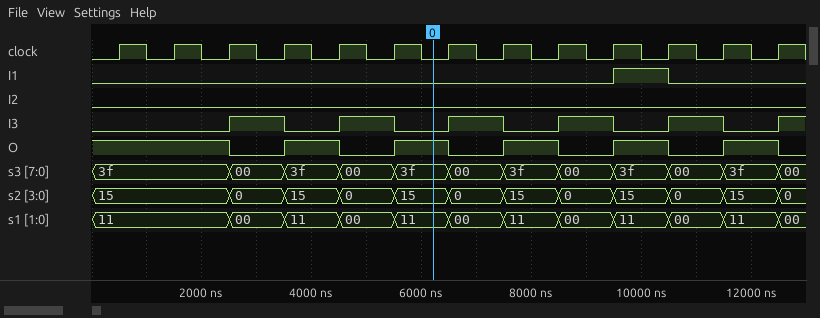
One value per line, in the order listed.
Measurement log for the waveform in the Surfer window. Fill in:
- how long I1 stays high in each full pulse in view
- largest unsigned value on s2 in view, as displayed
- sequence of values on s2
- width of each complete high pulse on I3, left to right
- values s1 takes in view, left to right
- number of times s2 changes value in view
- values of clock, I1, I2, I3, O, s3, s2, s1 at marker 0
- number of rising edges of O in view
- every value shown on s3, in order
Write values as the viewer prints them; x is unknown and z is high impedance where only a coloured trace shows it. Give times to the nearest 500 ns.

1000 ns
15
15, 0, 15, 0, 15, 0, 15, 0, 15, 0, 15, 0
1000 ns, 1000 ns, 1000 ns, 1000 ns, 1000 ns
11, 00, 11, 00, 11, 00, 11, 00, 11, 00, 11, 00
11
clock=0, I1=0, I2=0, I3=0, O=1, s3=3f, s2=15, s1=11
5
3f, 00, 3f, 00, 3f, 00, 3f, 00, 3f, 00, 3f, 00
